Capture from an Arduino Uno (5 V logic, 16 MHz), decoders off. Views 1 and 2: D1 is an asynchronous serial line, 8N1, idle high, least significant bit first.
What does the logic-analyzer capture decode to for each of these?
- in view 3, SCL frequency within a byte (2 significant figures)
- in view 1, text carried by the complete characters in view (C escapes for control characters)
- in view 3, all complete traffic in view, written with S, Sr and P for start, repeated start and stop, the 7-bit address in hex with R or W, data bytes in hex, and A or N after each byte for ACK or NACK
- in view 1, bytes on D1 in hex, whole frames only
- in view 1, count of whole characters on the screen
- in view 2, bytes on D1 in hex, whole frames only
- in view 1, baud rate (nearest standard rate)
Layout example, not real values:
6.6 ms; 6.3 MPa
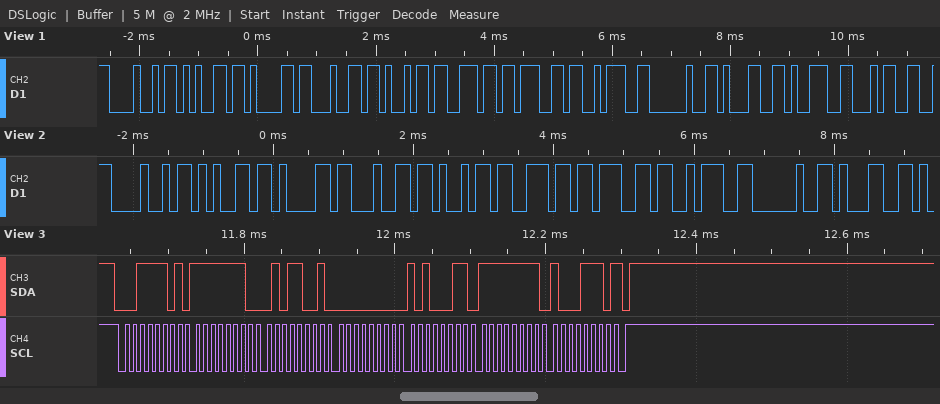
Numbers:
100 kHz; "Heading: 194"; S 1ER A FE A 59 A 00 A A3 A FF A 8E N P; 48 65 61 64 69 6E 67 3A 20 31 39 34; 12; 0x48 0x65 0x61 0x64 0x69 0x6E 0x67 0x3A 0x20 0x31; 9600 baud
